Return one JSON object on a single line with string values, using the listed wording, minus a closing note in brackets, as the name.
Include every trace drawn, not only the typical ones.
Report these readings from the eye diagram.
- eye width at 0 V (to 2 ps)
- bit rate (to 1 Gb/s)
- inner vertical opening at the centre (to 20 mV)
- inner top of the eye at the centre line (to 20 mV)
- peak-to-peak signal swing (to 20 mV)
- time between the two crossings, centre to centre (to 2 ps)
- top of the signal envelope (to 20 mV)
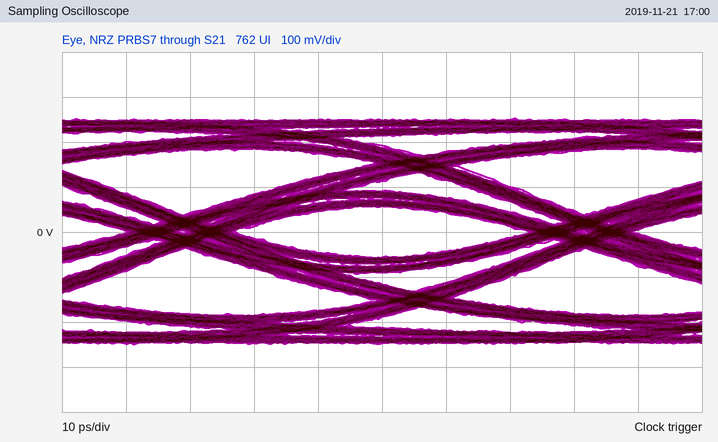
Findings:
{"eye width at 0 V": "46 ps", "bit rate": "16 Gb/s", "inner vertical opening at the centre": "120 mV", "inner top of the eye at the centre line": "60 mV", "peak-to-peak signal swing": "500 mV", "time between the two crossings, centre to centre": "62 ps", "top of the signal envelope": "260 mV"}
